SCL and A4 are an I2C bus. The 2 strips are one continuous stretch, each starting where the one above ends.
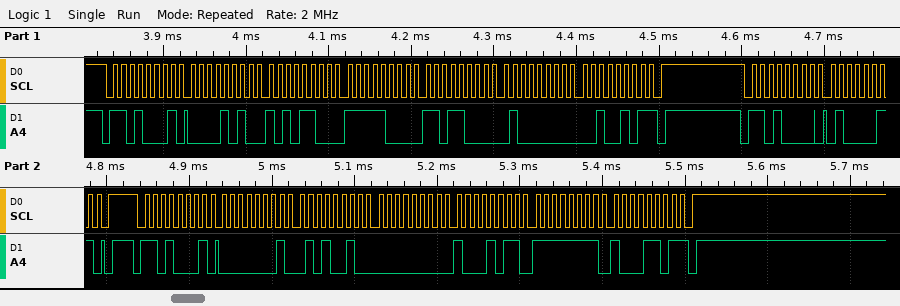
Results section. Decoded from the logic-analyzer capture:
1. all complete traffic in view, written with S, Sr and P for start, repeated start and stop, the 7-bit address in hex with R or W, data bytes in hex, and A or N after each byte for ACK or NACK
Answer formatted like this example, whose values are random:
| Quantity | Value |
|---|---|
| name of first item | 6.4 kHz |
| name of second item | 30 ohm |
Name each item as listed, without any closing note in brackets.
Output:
| Quantity | Value |
|---|---|
| all complete traffic in view, written with S, Sr and P for start, repeated start and stop, the 7-bit address in hex with R or W, data bytes in hex, and A or N after each byte for ACK or NACK | S 68R A 0A A AC A F8 A D8 A 40 A 25 N P S 68W A 43 A P S 68R A 01 A 52 A 00 A 8B A FF A 8D N P |
